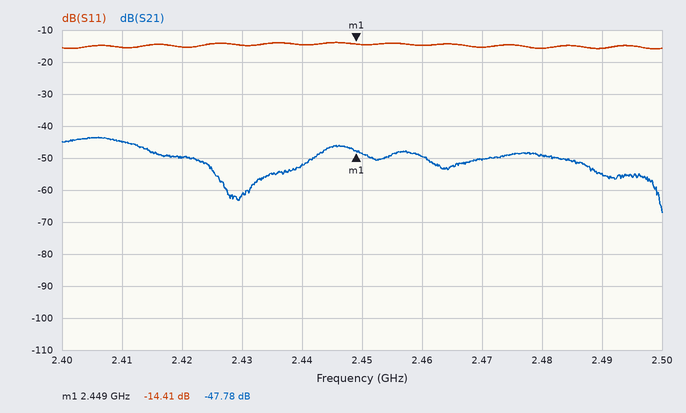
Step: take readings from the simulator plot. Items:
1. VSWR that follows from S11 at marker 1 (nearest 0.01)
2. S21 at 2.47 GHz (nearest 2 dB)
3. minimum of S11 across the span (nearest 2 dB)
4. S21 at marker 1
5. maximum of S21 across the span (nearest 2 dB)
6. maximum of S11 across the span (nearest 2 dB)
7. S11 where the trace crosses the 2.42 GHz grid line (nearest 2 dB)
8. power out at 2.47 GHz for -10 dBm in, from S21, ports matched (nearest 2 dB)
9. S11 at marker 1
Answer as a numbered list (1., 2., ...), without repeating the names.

1. 1.47
2. -50 dB
3. -16 dB
4. -47.78 dB
5. -44 dB
6. -14 dB
7. -16 dB
8. -60 dBm
9. -14.41 dB
